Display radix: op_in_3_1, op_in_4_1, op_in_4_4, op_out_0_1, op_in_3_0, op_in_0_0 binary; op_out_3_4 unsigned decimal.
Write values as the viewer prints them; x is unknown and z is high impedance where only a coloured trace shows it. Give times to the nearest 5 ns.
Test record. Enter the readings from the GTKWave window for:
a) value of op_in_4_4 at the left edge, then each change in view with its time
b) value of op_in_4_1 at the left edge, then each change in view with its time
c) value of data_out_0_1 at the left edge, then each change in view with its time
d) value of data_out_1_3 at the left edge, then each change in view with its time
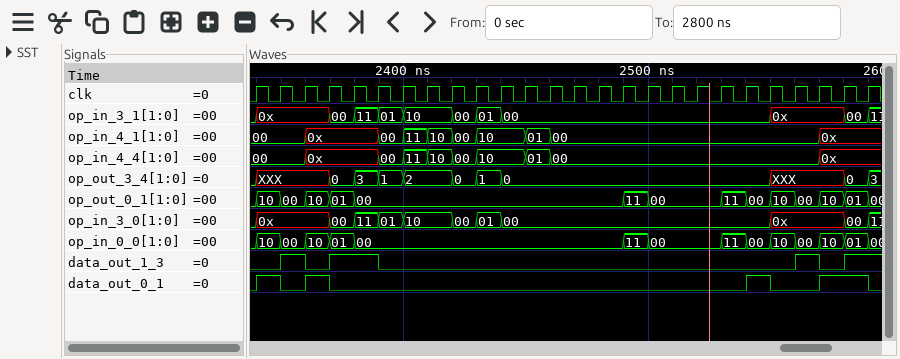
00, 0x at 2360 ns, 00 at 2390 ns, 11 at 2400 ns, 10 at 2410 ns, 00 at 2420 ns, 10 at 2430 ns, 01 at 2450 ns, 00 at 2460 ns, 0x at 2570 ns
00, 0x at 2360 ns, 00 at 2390 ns, 11 at 2400 ns, 10 at 2410 ns, 00 at 2420 ns, 10 at 2430 ns, 01 at 2450 ns, 00 at 2460 ns, 0x at 2570 ns
0, 1 at 2340 ns, 0 at 2350 ns, 1 at 2360 ns, 0 at 2370 ns, 1 at 2540 ns, 0 at 2550 ns, 1 at 2570 ns, 0 at 2590 ns
0, 1 at 2350 ns, 0 at 2360 ns, 1 at 2370 ns, 0 at 2390 ns, 1 at 2560 ns, 0 at 2570 ns, 1 at 2580 ns
